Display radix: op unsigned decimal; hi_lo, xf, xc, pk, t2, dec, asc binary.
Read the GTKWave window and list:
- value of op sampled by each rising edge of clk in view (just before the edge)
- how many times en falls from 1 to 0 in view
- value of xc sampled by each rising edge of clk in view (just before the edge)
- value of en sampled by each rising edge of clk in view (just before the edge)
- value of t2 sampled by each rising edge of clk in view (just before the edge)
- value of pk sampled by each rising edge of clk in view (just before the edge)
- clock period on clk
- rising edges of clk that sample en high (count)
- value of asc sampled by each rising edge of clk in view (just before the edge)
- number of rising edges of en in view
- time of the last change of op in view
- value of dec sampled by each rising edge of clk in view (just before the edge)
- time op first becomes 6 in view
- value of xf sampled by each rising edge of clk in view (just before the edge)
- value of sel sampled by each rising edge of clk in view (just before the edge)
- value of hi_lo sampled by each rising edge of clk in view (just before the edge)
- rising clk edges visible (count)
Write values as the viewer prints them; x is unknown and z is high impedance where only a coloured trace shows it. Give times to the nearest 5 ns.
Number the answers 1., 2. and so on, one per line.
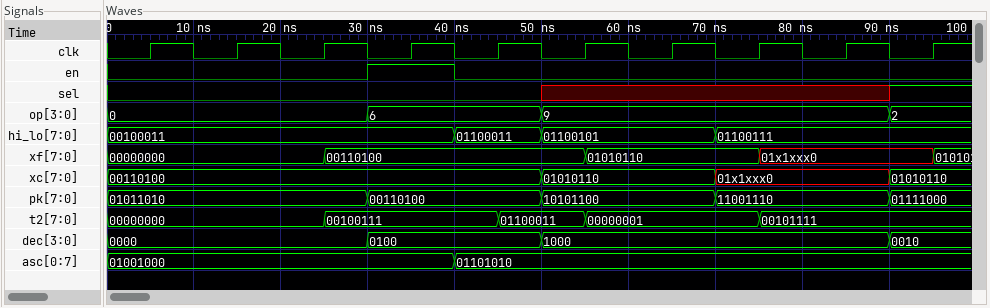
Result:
1. 0, 0, 0, 6, 6, 9, 9, 9, 9, 2
2. 1
3. 00110100, 00110100, 00110100, 00110100, 00110100, 01010110, 01010110, 01x1xxx0, 01x1xxx0, 01010110
4. 0 0 0 1 0 0 0 0 0 0
5. 00000000, 00000000, 00000000, 00100111, 00100111, 01100011, 00000001, 00000001, 00101111, 00101111
6. 01011010, 01011010, 01011010, 00110100, 00110100, 10101100, 10101100, 11001110, 11001110, 01111000
7. 10 ns
8. 1
9. 01001000, 01001000, 01001000, 01001000, 01101010, 01101010, 01101010, 01101010, 01101010, 01101010
10. 1
11. 90 ns
12. 0000, 0000, 0000, 0100, 0100, 1000, 1000, 1000, 1000, 0010
13. 30 ns
14. 00000000, 00000000, 00000000, 00110100, 00110100, 00110100, 01010110, 01010110, 01x1xxx0, 01x1xxx0
15. 0 0 0 0 0 x x x x 1
16. 00100011, 00100011, 00100011, 00100011, 01100011, 01100101, 01100101, 01100111, 01100111, 01100111
17. 10
